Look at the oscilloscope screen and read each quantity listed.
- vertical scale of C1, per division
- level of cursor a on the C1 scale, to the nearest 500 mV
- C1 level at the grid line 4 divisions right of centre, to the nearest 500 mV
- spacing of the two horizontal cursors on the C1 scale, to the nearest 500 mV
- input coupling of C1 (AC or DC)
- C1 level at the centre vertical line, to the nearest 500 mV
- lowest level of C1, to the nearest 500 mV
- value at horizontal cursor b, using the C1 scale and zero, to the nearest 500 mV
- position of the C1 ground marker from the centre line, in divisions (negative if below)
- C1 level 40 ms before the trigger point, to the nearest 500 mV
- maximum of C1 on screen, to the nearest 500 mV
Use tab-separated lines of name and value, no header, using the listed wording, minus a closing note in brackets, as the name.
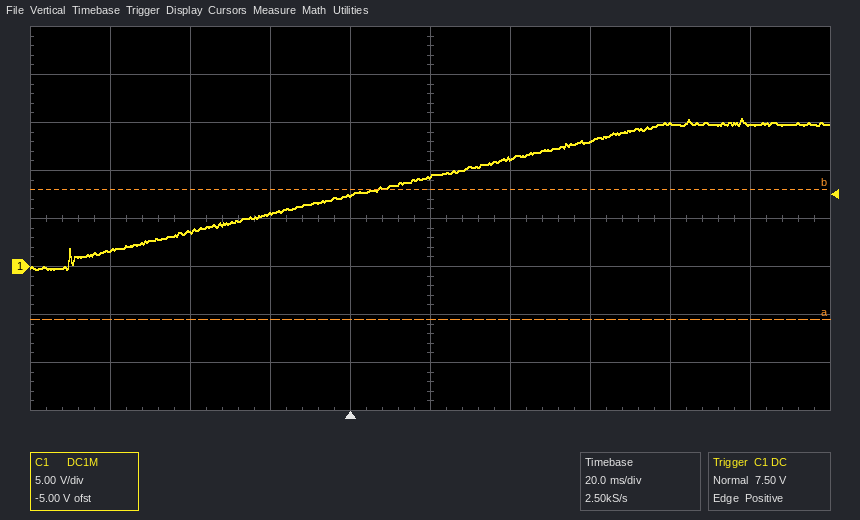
vertical scale of C1, per division	5 V
level of cursor a on the C1 scale, to the nearest 500 mV	-5.5 V
C1 level at the grid line 4 divisions right of centre, to the nearest 500 mV	15.0 V
spacing of the two horizontal cursors on the C1 scale, to the nearest 500 mV	13.5 V
input coupling of C1	DC
C1 level at the centre vertical line, to the nearest 500 mV	9.5 V
lowest level of C1, to the nearest 500 mV	-500 mV
value at horizontal cursor b, using the C1 scale and zero, to the nearest 500 mV	8.0 V
position of the C1 ground marker from the centre line, in divisions	-1.0 div
C1 level 40 ms before the trigger point, to the nearest 500 mV	3.5 V
maximum of C1 on screen, to the nearest 500 mV	15.5 V
